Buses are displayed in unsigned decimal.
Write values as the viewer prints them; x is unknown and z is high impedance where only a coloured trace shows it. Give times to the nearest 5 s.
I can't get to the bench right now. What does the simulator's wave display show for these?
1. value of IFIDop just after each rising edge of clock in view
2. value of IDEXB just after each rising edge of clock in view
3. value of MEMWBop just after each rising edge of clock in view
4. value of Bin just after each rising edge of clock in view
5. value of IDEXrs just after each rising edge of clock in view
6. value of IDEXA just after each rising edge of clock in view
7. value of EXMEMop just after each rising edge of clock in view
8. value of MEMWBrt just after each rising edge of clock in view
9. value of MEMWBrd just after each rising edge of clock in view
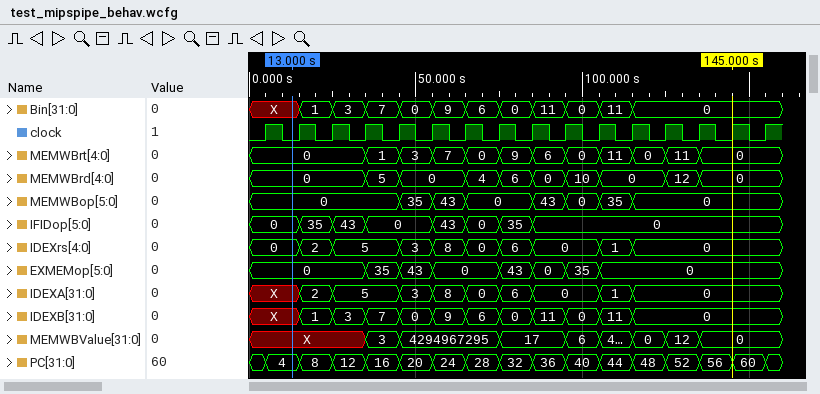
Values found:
0, 35, 43, 0, 0, 43, 0, 35, 0, 0, 0, 0, 0, 0, 0, 0
X, 1, 3, 7, 0, 9, 6, 0, 11, 0, 11, 0, 0, 0, 0, 0
0, 0, 0, 0, 35, 43, 0, 0, 43, 0, 35, 0, 0, 0, 0, 0
X, 1, 3, 7, 0, 9, 6, 0, 11, 0, 11, 0, 0, 0, 0, 0
0, 2, 5, 5, 3, 8, 0, 6, 0, 0, 1, 0, 0, 0, 0, 0
X, 2, 5, 5, 3, 8, 0, 6, 0, 0, 1, 0, 0, 0, 0, 0
0, 0, 0, 35, 43, 0, 0, 43, 0, 35, 0, 0, 0, 0, 0, 0
0, 0, 0, 1, 3, 7, 0, 9, 6, 0, 11, 0, 11, 0, 0, 0
0, 0, 0, 5, 0, 0, 4, 6, 0, 10, 0, 0, 12, 0, 0, 0
